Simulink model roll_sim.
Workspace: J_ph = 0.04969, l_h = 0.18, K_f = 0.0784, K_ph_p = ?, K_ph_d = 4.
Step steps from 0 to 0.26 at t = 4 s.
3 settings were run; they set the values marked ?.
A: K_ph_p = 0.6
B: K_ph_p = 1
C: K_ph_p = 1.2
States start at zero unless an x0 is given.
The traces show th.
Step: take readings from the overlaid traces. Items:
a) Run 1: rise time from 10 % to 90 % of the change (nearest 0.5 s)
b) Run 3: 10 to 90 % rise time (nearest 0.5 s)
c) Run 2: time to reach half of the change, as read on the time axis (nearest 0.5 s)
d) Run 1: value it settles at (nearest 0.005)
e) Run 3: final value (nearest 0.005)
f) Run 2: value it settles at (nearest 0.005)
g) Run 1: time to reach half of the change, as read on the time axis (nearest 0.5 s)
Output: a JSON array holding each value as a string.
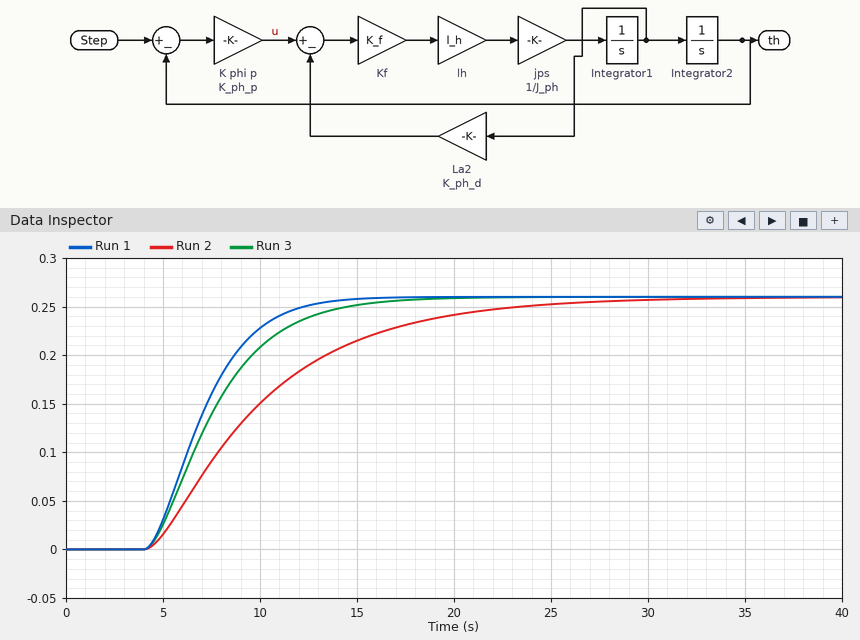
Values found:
["5.5 s", "7.0 s", "9.0 s", "0.260", "0.260", "0.260", "7.0 s"]
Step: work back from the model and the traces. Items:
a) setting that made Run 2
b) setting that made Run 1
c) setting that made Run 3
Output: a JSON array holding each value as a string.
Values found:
["A", "C", "B"]
